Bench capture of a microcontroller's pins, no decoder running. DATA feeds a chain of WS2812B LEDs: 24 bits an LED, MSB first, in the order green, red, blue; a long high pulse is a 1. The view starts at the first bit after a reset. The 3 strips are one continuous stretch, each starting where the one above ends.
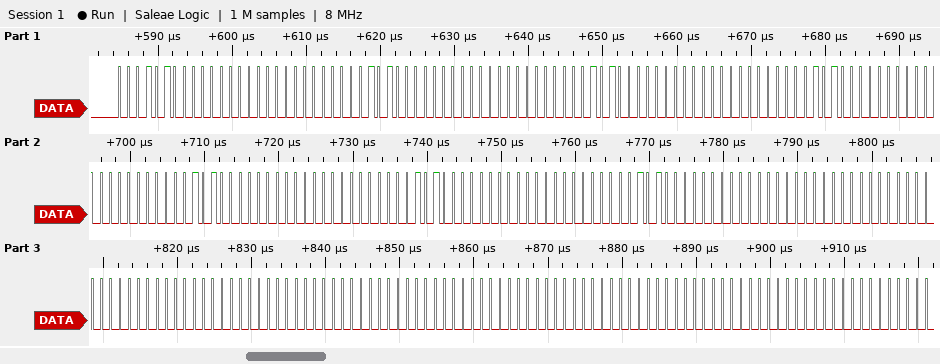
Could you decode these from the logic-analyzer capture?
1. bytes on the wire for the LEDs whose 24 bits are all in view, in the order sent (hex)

14 00 00 14 00 00 14 00 00 14 00 00 14 00 00 14 00 00 14 00 00 00 00 00 00 00 00 00 00 00 00 00 00
